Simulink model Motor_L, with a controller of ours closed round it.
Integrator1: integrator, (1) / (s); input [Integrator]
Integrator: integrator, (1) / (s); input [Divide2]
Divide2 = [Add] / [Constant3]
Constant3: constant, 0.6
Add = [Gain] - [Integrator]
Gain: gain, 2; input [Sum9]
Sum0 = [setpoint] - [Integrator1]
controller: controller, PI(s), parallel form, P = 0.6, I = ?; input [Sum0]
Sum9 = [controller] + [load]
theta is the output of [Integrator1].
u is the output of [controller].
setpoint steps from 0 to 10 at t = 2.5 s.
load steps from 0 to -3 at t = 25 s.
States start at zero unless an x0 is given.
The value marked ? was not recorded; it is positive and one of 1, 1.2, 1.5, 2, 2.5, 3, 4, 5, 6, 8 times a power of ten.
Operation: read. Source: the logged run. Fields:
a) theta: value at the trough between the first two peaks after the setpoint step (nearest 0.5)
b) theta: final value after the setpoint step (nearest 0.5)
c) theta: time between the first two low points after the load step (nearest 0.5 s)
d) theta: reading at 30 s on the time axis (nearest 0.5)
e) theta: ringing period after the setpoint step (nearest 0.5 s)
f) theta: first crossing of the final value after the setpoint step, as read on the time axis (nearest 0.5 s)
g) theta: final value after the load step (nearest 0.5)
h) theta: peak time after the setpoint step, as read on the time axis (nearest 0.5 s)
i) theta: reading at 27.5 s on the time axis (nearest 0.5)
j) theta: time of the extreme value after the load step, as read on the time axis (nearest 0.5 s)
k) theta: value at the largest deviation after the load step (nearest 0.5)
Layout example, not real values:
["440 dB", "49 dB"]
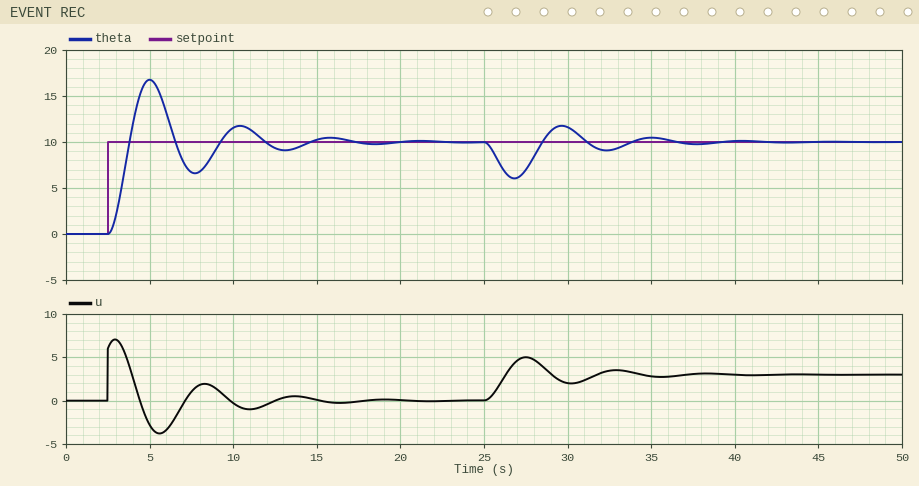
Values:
["6.5", "10.0", "5.5 s", "11.5", "5.5 s", "4.0 s", "10.0", "5.0 s", "7.0", "27.0 s", "6.0"]
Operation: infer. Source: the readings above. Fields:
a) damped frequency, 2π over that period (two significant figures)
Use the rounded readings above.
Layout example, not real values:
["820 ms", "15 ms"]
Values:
["1.1 rad/s"]
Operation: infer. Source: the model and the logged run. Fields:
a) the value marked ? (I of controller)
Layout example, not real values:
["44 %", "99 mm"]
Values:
["0.5"]
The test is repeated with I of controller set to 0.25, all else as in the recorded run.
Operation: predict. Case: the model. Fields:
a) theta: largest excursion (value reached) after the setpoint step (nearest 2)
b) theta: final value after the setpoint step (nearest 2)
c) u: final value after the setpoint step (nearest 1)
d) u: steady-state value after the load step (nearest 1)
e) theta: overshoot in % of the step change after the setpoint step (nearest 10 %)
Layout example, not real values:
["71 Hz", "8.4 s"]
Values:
["14", "10", "0", "3", "40 %"]
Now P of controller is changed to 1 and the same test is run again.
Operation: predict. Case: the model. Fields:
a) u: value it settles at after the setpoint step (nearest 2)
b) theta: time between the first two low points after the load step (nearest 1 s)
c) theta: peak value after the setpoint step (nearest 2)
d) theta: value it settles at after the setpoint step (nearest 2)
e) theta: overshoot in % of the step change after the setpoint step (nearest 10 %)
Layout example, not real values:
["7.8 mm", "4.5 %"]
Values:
["0", "4 s", "16", "10", "50 %"]
